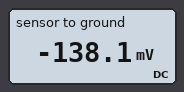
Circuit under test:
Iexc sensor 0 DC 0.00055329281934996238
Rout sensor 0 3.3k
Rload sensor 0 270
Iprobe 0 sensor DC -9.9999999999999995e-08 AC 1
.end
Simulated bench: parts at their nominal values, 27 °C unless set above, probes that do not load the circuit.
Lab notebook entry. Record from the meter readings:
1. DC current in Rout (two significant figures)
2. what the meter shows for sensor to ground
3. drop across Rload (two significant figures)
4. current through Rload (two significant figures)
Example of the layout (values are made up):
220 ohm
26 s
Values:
42 µA
-138.1 mV
140 mV
510 µA
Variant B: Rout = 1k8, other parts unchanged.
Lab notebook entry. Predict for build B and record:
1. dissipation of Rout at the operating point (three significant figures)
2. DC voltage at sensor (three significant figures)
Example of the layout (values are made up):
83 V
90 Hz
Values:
9.38 µW
-130 mV
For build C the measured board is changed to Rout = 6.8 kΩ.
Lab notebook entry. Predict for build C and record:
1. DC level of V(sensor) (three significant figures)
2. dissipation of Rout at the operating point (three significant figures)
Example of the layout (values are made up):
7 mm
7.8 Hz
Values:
-144 mV
3.04 µW
